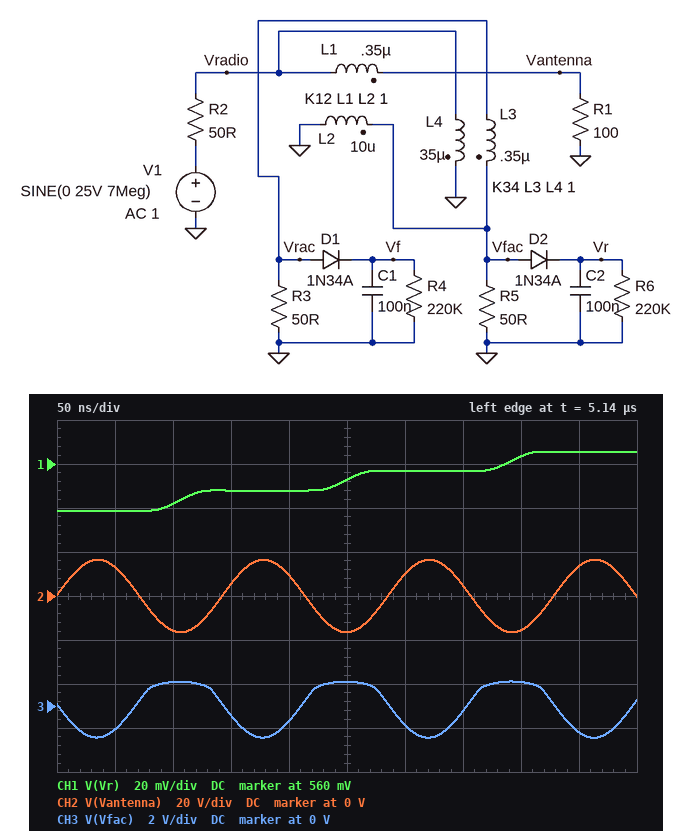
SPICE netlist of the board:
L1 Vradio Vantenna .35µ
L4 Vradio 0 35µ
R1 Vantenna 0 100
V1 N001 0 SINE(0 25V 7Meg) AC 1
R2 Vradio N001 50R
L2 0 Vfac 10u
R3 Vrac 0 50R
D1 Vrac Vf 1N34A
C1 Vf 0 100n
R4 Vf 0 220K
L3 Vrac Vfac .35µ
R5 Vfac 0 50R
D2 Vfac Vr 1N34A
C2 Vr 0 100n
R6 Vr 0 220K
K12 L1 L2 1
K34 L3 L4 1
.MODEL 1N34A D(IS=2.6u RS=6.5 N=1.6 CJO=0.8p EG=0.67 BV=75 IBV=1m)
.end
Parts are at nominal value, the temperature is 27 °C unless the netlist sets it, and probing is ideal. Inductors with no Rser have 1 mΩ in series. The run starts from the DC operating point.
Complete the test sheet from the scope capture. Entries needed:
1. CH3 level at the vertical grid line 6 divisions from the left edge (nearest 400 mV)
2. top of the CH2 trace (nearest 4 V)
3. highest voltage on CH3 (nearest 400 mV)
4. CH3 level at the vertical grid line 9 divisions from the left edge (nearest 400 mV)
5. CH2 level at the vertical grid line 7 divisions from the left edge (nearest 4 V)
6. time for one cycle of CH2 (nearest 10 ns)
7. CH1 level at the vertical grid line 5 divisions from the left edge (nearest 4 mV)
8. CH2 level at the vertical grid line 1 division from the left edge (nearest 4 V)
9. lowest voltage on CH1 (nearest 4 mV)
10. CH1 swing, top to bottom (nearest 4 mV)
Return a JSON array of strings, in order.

["-800 mV", "16 V", "1.2 V", "-1.2 V", "4 V", "140 ns", "552 mV", "12 V", "540 mV", "28 mV"]
